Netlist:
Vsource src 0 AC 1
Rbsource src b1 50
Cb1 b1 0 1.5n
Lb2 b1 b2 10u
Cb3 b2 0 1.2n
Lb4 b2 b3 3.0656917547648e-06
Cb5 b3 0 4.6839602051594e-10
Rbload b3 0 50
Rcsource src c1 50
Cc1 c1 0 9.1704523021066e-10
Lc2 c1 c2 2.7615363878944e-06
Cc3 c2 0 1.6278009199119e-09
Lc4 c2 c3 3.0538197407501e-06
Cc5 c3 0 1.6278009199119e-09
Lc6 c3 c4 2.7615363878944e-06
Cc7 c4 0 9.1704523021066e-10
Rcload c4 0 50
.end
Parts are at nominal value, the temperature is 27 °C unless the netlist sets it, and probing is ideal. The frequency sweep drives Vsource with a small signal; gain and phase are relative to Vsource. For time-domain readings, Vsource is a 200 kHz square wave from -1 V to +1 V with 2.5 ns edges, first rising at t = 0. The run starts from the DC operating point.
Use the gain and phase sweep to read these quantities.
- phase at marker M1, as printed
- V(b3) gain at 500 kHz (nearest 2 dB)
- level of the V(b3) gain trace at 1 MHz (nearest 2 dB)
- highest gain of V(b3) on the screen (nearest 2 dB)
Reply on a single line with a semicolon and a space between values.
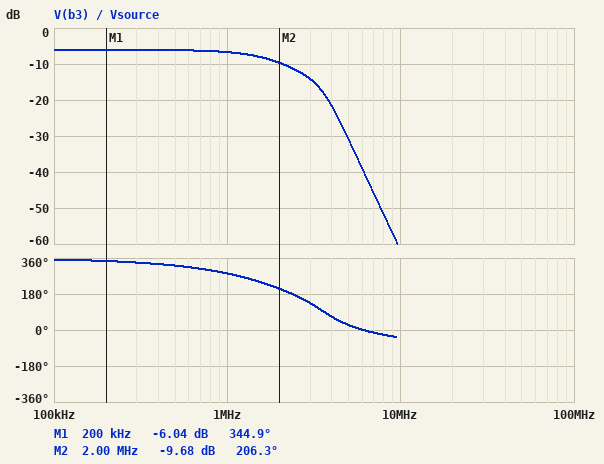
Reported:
344.9 deg; -6 dB; -6 dB; -6 dB
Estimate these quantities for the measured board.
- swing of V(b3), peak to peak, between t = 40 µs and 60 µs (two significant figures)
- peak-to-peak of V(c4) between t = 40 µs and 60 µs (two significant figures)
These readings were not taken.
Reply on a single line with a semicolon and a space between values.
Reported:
1.0 V; 1.4 V
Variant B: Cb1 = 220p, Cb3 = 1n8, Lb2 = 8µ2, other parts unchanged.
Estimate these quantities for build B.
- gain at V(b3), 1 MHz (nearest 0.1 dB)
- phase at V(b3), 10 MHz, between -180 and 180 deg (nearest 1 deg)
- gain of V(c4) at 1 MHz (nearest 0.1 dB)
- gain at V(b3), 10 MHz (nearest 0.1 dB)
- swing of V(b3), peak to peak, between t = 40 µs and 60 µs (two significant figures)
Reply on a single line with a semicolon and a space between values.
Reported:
-6.5 dB; 9 deg; -6.1 dB; -51.6 dB; 1.1 V
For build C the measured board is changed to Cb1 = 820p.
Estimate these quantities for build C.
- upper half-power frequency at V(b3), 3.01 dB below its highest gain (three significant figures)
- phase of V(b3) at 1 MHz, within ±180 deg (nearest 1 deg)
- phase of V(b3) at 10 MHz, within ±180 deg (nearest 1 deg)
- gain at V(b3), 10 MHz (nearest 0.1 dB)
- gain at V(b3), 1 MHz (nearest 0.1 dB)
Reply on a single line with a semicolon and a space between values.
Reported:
2.08 MHz; -69 deg; -28 deg; -56.8 dB; -6.8 dB
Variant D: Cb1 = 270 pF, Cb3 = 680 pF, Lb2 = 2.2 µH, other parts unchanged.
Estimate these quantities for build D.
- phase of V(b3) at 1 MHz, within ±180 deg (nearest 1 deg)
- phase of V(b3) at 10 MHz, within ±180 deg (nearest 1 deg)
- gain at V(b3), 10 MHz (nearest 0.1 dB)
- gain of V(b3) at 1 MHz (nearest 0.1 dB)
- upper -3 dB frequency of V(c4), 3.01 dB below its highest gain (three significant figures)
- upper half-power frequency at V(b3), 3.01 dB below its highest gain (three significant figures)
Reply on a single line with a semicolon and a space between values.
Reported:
-32 deg; 19 deg; -28.5 dB; -6.1 dB; 4.38 MHz; 6.44 MHz
